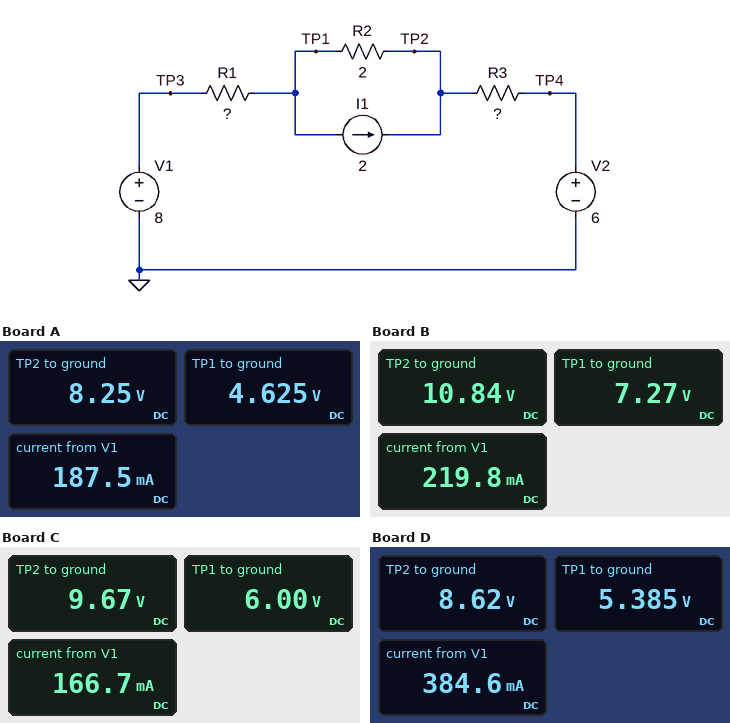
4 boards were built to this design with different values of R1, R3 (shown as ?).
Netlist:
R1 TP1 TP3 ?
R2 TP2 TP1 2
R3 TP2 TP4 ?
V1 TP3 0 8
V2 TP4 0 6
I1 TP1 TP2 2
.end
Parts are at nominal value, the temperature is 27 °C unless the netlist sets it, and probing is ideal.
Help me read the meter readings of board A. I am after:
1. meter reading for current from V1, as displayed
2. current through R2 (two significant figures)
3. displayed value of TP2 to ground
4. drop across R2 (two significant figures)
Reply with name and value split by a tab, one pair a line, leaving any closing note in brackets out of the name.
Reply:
meter reading for current from V1, as displayed	187.5 mA
current through R2	1.8 A
displayed value of TP2 to ground	8.25 V
drop across R2	3.6 V
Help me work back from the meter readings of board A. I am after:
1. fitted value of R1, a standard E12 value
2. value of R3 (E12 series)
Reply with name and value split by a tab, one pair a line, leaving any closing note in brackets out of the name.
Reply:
fitted value of R1, a standard E12 value	18 Ω
value of R3	12 Ω
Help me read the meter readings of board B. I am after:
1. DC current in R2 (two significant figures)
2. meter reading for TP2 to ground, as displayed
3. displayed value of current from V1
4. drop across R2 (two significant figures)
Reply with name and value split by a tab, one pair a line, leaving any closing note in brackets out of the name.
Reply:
DC current in R2	1.8 A
meter reading for TP2 to ground, as displayed	10.84 V
displayed value of current from V1	219.8 mA
drop across R2	3.6 V
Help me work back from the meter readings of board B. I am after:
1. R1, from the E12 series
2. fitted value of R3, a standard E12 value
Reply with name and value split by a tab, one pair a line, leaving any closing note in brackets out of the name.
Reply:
R1, from the E12 series	3.3 Ω
fitted value of R3, a standard E12 value	22 Ω
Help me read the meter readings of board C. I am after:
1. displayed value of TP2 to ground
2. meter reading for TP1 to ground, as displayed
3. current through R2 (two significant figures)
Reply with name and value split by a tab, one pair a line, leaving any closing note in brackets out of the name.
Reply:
displayed value of TP2 to ground	9.67 V
meter reading for TP1 to ground, as displayed	6.00 V
current through R2	1.8 A
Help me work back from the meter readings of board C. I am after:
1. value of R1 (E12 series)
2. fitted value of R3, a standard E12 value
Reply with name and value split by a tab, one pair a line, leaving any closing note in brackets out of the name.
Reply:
value of R1	12 Ω
fitted value of R3, a standard E12 value	22 Ω
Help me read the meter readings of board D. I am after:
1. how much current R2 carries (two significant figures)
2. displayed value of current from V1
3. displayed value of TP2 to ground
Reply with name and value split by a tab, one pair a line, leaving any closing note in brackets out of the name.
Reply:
how much current R2 carries	1.6 A
displayed value of current from V1	384.6 mA
displayed value of TP2 to ground	8.62 V
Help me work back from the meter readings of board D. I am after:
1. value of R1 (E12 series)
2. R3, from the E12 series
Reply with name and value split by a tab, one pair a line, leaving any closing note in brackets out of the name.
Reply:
value of R1	6.8 Ω
R3, from the E12 series	6.8 Ω
